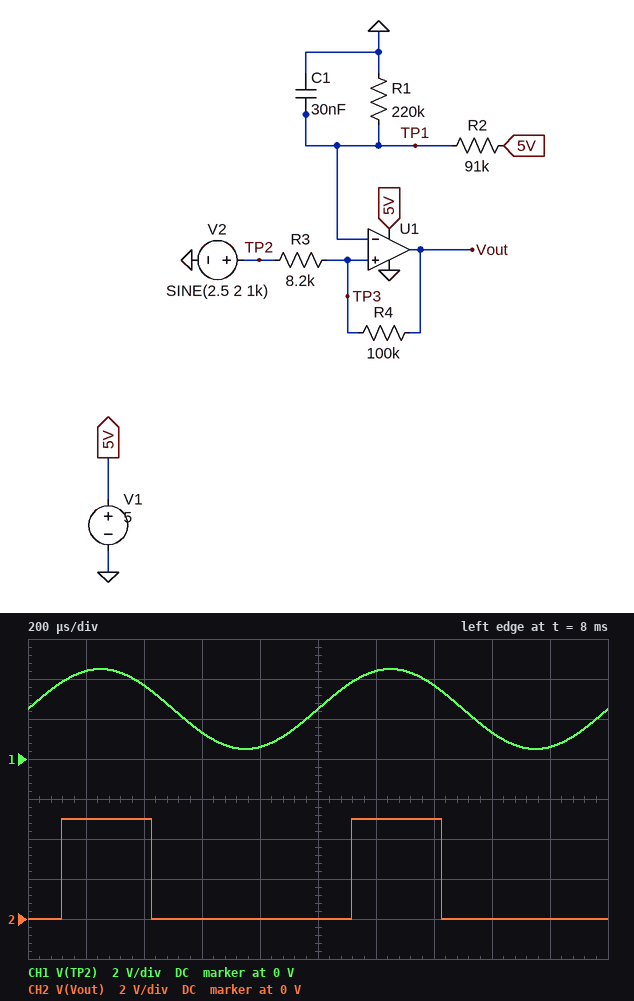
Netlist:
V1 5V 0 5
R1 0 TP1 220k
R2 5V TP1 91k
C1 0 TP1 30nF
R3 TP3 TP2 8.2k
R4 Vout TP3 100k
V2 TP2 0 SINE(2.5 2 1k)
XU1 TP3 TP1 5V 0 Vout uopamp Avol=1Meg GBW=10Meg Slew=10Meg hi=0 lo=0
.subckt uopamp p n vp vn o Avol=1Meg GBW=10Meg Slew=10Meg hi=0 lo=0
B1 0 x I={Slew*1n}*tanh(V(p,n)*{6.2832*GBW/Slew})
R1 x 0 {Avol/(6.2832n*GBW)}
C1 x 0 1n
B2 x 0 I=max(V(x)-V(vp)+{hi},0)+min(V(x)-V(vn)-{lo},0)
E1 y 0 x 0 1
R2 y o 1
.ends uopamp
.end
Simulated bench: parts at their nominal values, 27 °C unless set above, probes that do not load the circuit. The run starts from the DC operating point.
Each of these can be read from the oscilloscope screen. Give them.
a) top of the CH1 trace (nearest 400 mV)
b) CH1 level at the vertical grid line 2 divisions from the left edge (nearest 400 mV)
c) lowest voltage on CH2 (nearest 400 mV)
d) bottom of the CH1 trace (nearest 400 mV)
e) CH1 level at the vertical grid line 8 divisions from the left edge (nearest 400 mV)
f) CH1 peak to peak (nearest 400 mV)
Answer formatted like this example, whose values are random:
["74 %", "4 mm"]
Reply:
["4.4 V", "3.6 V", "0 V", "400 mV", "1.2 V", "4.0 V"]
